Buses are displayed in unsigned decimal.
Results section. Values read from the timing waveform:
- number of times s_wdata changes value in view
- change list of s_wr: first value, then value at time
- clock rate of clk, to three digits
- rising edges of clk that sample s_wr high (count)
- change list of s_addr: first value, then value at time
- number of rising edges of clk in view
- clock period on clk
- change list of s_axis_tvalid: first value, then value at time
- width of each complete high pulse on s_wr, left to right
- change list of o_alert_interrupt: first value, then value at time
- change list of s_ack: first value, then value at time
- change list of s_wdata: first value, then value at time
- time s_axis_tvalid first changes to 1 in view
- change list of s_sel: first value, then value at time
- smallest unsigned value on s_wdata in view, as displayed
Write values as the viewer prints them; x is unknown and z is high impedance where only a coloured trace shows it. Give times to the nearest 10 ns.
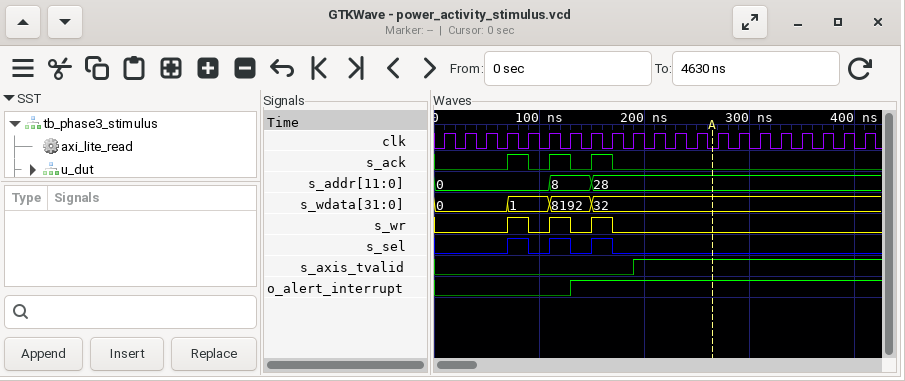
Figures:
3
0, 1 at 70 ns, 0 at 90 ns, 1 at 110 ns, 0 at 130 ns, 1 at 150 ns, 0 at 170 ns
50.0 MHz
3
0, 8 at 110 ns, 28 at 150 ns
21
20 ns
0, 1 at 190 ns
20 ns, 20 ns, 20 ns
0, 1 at 130 ns
0, 1 at 70 ns, 0 at 90 ns, 1 at 110 ns, 0 at 130 ns, 1 at 150 ns, 0 at 170 ns
0, 1 at 70 ns, 8192 at 110 ns, 32 at 150 ns
190 ns
0, 1 at 70 ns, 0 at 90 ns, 1 at 110 ns, 0 at 130 ns, 1 at 150 ns, 0 at 170 ns
0
